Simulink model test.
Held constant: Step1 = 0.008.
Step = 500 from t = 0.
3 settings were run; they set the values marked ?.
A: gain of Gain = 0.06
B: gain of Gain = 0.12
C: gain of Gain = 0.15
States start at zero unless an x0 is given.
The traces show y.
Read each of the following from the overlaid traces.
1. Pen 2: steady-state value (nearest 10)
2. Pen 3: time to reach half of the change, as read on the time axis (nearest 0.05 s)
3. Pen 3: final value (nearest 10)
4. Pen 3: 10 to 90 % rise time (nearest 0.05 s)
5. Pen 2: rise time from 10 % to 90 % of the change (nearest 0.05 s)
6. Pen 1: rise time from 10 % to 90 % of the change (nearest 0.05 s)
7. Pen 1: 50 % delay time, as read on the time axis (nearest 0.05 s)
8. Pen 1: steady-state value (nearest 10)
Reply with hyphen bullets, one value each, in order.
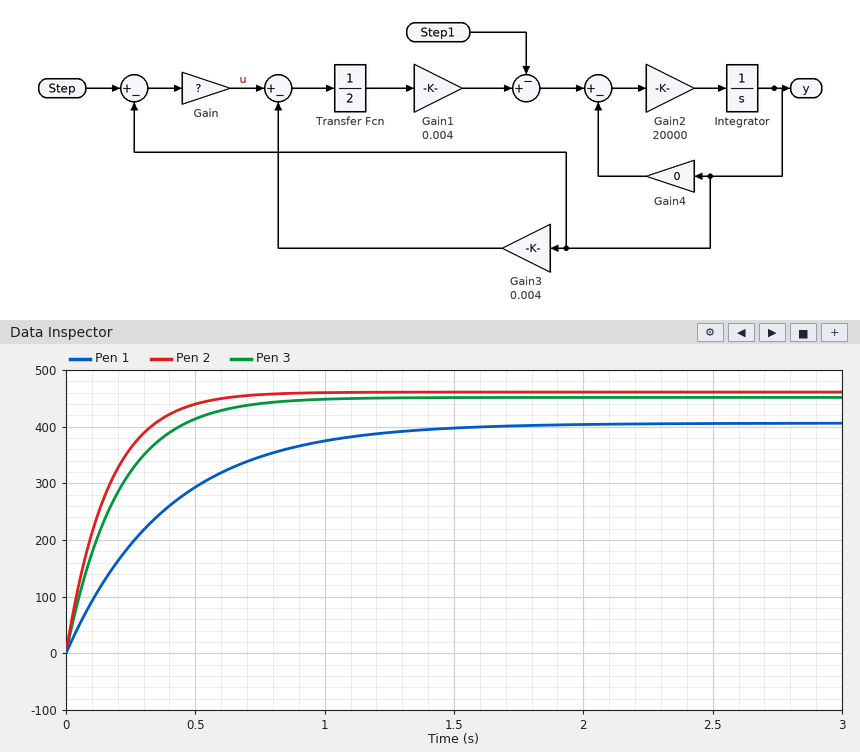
- 460
- 0.15 s
- 450
- 0.45 s
- 0.35 s
- 0.85 s
- 0.25 s
- 410
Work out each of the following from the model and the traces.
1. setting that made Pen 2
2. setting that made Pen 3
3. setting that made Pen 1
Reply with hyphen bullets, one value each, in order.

- C
- B
- A
